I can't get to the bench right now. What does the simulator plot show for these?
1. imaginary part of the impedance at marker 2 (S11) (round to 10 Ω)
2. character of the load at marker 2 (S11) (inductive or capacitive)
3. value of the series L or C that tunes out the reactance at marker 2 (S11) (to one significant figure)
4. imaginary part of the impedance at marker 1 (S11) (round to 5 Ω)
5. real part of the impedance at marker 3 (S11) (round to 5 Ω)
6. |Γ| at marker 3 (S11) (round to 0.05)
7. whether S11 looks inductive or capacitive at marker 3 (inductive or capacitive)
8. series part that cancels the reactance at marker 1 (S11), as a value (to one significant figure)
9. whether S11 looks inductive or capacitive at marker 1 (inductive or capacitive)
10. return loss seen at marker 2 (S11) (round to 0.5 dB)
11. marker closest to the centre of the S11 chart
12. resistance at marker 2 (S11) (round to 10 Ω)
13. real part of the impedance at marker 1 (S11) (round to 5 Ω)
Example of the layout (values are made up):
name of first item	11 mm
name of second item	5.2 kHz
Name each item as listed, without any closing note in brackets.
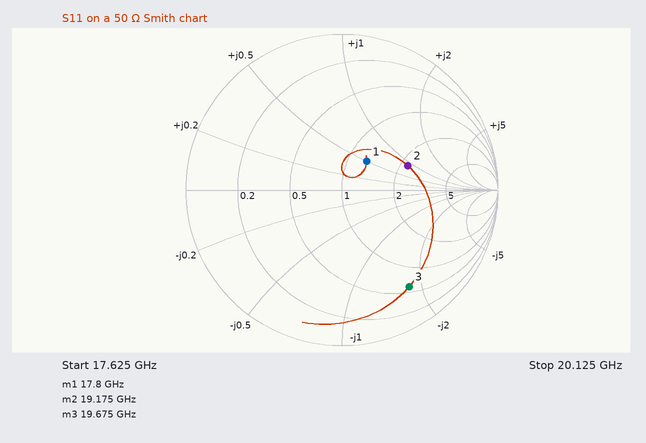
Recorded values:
imaginary part of the impedance at marker 2 (S11)	+40 Ω
character of the load at marker 2 (S11)	inductive
value of the series L or C that tunes out the reactance at marker 2 (S11)	200 fF
imaginary part of the impedance at marker 1 (S11)	+25 Ω
real part of the impedance at marker 3 (S11)	30 Ω
|Γ| at marker 3 (S11)	0.75
whether S11 looks inductive or capacitive at marker 3	capacitive
series part that cancels the reactance at marker 1 (S11), as a value	400 fF
whether S11 looks inductive or capacitive at marker 1	inductive
return loss seen at marker 2 (S11)	7.0 dB
marker closest to the centre of the S11 chart	marker 1
resistance at marker 2 (S11)	110 Ω
real part of the impedance at marker 1 (S11)	65 Ω
